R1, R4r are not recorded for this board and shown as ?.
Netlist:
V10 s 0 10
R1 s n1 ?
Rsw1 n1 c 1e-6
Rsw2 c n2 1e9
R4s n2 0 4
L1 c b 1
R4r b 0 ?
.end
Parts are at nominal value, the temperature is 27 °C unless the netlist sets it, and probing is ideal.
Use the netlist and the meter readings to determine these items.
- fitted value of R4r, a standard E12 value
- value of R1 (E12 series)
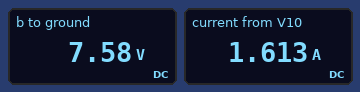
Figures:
4.7 Ω
1.5 Ω
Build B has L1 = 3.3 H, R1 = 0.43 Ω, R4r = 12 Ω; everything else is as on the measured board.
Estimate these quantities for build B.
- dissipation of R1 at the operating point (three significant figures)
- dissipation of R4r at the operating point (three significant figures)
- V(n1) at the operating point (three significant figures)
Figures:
278 mW
7.77 W
9.65 V
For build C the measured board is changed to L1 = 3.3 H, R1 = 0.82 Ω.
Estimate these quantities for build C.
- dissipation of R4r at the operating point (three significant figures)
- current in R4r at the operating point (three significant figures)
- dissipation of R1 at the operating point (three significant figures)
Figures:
15.4 W
1.81 A
2.69 W
